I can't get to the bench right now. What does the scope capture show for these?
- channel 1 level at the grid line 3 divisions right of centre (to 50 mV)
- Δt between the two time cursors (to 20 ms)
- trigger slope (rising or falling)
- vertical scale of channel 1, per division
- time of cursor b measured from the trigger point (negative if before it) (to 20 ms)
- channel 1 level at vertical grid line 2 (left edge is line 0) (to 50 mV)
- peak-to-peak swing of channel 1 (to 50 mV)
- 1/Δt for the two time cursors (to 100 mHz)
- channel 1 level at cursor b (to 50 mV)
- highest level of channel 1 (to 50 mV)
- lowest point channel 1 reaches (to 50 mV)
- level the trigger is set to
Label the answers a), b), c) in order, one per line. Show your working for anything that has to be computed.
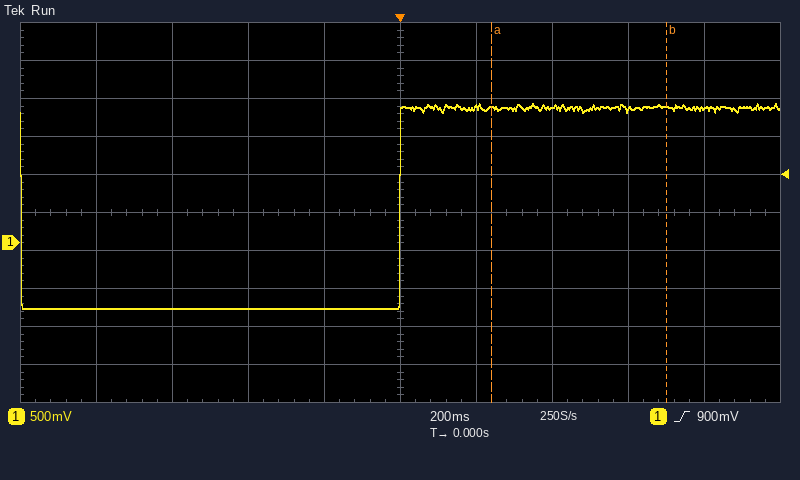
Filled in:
a) 1.75 V
b) 460 ms
c) rising
d) 500 mV
e) +700 ms
f) -850 mV
g) 1.85 V − (-850 mV) = 2.70 V
h) 1 / 460 ms ≈ 2.2 Hz
i) 1.80 V
j) 1.85 V
k) -850 mV
l) 900 mV
